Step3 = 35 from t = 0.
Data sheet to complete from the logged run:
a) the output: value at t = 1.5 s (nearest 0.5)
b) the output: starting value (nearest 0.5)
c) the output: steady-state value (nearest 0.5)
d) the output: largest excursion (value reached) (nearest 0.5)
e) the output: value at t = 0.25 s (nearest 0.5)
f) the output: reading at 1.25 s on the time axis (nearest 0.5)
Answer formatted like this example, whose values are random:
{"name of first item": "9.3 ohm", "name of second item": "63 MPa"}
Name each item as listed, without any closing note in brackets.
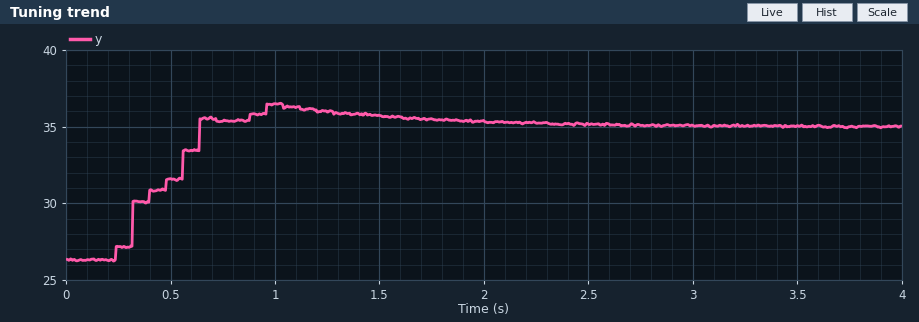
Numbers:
{"the output: value at t = 1.5 s": "35.5", "the output: starting value": "26.5", "the output: steady-state value": "35.0", "the output: largest excursion (value reached)": "36.5", "the output: value at t = 0.25 s": "27.0", "the output: reading at 1.25 s on the time axis": "36.0"}
